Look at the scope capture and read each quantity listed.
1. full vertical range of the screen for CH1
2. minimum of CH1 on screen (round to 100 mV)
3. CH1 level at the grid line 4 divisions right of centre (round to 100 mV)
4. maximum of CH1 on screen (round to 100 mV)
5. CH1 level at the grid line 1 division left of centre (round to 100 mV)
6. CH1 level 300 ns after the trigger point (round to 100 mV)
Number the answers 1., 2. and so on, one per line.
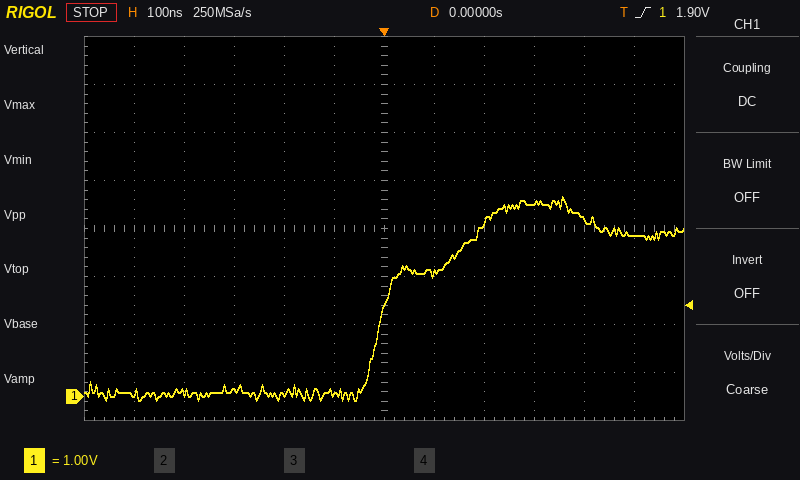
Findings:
1. 8 V
2. -100 mV
3. 3.7 V
4. 4.2 V
5. 100 mV
6. 4.0 V
